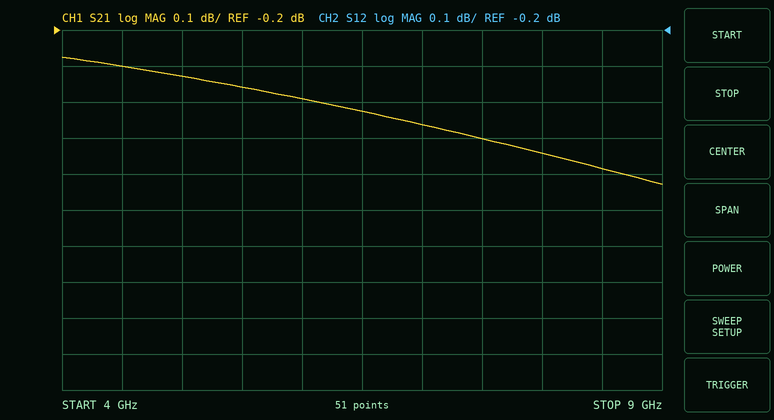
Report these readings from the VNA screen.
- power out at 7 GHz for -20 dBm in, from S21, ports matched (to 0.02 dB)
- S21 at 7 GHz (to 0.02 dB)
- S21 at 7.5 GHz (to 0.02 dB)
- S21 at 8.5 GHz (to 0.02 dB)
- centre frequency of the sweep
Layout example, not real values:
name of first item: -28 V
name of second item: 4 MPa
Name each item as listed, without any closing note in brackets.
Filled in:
power out at 7 GHz for -20 dBm in, from S21, ports matched: -20.46 dBm
S21 at 7 GHz: -0.46 dB
S21 at 7.5 GHz: -0.50 dB
S21 at 8.5 GHz: -0.58 dB
centre frequency of the sweep: 6.5 GHz
